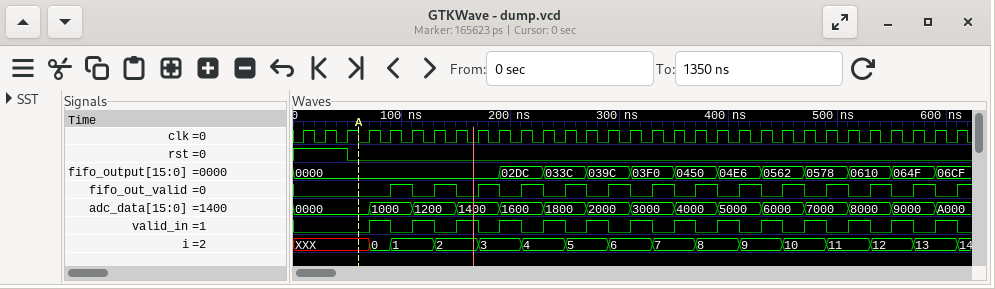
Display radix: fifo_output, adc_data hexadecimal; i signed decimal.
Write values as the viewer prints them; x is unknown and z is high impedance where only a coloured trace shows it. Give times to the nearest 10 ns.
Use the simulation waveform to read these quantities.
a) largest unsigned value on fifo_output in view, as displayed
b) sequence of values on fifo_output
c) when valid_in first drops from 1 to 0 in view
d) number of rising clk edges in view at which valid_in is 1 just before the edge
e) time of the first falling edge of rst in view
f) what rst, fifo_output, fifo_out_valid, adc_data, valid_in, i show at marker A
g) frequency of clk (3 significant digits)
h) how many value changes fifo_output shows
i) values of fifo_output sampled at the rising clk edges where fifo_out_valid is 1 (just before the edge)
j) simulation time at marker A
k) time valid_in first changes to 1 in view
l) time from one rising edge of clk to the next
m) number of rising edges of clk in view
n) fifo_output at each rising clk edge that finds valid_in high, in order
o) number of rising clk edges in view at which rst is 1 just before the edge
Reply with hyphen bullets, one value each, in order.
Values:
- 06CF
- 0000, 02DC, 033C, 039C, 03F0, 0450, 04E6, 0562, 0578, 0610, 064F, 06CF
- 90 ns
- 14
- 50 ns
- rst=0, fifo_output=0000, fifo_out_valid=0, adc_data=0000, valid_in=0, i=XXX
- 50.0 MHz
- 11
- 0000, 0000, 0000, 02DC, 033C, 039C, 03F0, 0450, 04E6, 0562, 0578, 0610, 064F
- 60 ns
- 70 ns
- 20 ns
- 31
- 0000, 0000, 0000, 02DC, 033C, 039C, 03F0, 0450, 04E6, 0562, 0578, 0610, 064F, 06CF
- 3
